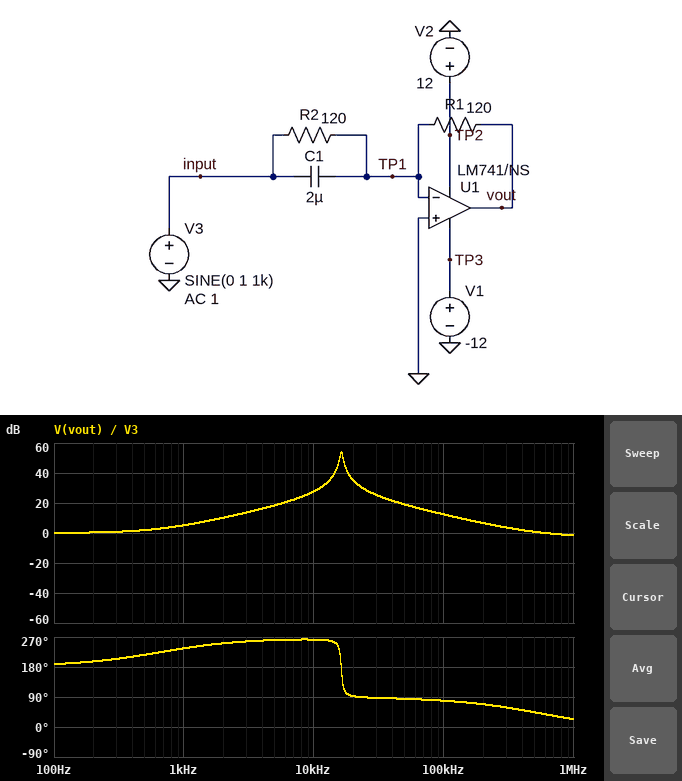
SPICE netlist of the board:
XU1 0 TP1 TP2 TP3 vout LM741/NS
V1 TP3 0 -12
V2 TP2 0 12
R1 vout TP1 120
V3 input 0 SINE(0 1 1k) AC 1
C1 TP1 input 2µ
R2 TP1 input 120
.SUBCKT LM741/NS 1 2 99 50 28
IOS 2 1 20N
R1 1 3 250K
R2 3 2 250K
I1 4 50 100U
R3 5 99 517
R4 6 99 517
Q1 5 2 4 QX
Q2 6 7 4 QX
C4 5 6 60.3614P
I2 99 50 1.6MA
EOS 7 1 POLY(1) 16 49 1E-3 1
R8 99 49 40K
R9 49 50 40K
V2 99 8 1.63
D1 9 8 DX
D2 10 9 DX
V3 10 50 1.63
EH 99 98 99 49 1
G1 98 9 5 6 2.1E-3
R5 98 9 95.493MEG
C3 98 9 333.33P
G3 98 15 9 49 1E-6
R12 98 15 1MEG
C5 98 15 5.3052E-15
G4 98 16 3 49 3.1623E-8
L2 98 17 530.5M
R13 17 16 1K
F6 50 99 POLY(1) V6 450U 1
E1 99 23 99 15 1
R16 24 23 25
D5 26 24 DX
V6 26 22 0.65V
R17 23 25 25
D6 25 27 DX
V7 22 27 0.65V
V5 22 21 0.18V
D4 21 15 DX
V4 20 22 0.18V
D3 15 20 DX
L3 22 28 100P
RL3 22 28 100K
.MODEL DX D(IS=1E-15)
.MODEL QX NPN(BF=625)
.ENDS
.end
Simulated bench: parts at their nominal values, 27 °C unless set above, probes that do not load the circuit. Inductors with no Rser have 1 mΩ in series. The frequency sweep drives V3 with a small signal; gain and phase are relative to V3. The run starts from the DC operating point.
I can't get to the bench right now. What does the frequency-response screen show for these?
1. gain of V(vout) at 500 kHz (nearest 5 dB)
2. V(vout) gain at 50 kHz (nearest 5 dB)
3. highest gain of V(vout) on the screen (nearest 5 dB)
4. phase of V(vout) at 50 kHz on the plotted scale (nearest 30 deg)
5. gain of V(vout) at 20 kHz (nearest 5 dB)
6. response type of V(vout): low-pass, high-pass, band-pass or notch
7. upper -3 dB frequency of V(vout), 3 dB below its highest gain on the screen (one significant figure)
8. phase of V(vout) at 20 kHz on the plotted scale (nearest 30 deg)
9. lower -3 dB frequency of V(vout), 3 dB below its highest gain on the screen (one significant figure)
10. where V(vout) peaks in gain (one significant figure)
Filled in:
0 dB
20 dB
55 dB
90 deg
35 dB
band-pass
20 kHz
90 deg
20 kHz
20 kHz
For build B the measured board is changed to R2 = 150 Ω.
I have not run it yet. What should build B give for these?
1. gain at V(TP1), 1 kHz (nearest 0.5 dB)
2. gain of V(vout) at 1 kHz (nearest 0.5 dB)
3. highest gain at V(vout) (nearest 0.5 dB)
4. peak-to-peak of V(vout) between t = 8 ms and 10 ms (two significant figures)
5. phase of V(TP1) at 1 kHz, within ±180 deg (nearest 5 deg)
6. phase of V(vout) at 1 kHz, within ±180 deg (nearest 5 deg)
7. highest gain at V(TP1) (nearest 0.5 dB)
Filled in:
-47.5 dB
4.5 dB
55.5 dB
3.5 V
150 deg
-120 deg
27.5 dB
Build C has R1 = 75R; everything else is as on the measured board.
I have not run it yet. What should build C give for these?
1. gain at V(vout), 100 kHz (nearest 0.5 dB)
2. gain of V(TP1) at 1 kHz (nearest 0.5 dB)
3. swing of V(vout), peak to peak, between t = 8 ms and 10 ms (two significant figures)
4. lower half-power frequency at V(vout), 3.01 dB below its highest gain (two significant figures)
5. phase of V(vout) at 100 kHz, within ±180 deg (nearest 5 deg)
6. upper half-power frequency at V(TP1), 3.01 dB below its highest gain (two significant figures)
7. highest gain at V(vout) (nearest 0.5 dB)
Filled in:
10.0 dB
-48.0 dB
2.3 V
17 kHz
75 deg
18 kHz
51.0 dB
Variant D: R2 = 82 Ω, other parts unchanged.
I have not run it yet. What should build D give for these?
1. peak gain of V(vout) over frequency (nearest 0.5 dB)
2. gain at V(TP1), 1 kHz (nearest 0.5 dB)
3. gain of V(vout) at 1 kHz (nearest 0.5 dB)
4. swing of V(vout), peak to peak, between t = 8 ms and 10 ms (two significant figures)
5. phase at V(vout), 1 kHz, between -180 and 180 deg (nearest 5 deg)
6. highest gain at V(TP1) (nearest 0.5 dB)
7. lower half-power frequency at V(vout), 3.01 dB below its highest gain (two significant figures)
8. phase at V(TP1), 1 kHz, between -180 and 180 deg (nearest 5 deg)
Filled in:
51.0 dB
-45.5 dB
6.5 dB
4.3 V
-135 deg
23.5 dB
16 kHz
135 deg
